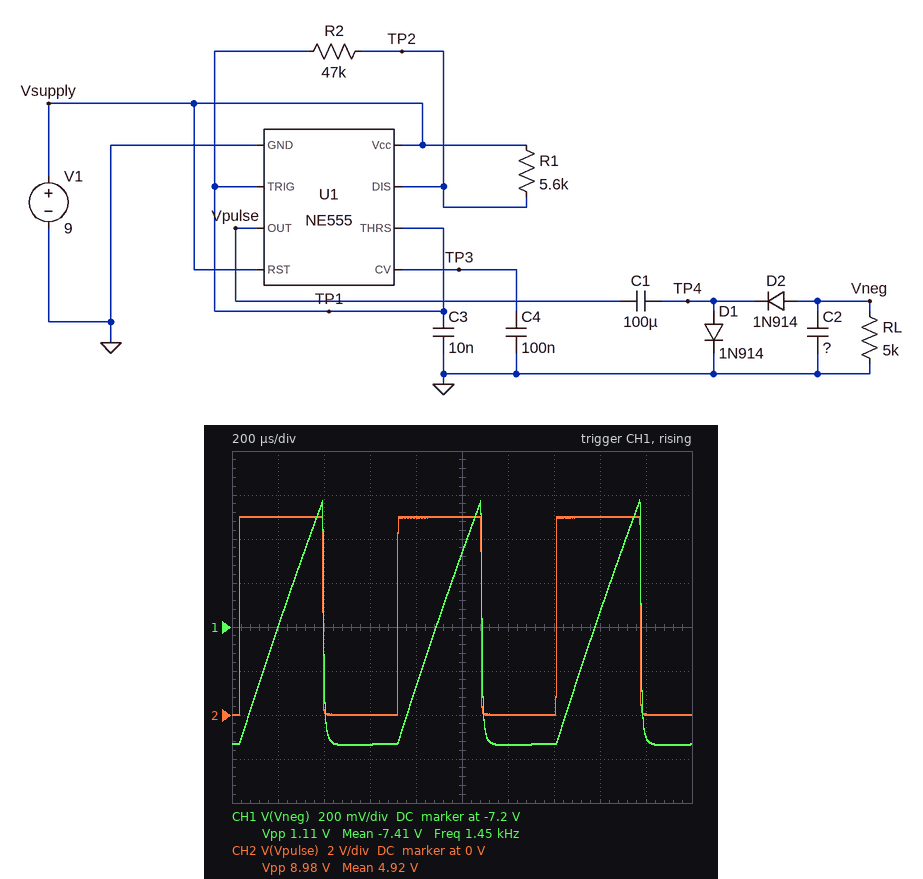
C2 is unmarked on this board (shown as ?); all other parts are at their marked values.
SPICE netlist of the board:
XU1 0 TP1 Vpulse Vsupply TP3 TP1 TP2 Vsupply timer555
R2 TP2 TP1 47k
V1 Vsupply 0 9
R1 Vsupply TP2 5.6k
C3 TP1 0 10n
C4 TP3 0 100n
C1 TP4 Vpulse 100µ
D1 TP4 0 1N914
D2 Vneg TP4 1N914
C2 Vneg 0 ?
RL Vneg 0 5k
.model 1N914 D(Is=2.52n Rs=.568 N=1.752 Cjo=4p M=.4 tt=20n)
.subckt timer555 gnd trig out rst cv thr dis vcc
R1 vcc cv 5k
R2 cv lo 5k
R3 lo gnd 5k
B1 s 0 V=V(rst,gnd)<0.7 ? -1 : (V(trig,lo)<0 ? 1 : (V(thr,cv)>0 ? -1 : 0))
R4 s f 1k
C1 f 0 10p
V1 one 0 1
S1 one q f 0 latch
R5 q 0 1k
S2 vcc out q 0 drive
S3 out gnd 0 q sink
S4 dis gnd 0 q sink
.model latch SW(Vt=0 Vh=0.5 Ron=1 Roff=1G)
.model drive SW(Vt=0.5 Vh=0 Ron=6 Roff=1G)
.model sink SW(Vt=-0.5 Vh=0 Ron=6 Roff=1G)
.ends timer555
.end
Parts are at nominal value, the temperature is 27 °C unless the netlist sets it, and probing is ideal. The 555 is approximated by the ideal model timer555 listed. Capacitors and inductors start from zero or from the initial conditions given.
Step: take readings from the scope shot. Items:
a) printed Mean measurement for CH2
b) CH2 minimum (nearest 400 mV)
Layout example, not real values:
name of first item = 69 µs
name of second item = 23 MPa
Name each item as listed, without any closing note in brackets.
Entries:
printed Mean measurement for CH2 = 4.92 V
CH2 minimum = 0 V
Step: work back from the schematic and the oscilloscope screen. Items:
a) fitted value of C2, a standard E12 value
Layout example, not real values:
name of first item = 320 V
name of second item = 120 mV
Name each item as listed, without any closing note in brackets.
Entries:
fitted value of C2, a standard E12 value = 470 nF
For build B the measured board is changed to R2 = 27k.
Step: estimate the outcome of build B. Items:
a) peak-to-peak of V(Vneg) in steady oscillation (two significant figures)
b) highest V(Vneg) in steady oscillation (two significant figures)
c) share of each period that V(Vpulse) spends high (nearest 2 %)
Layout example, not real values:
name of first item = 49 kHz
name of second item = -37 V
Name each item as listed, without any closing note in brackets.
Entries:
peak-to-peak of V(Vneg) in steady oscillation = 710 mV
highest V(Vneg) in steady oscillation = -7.0 V
share of each period that V(Vpulse) spends high = 54 %
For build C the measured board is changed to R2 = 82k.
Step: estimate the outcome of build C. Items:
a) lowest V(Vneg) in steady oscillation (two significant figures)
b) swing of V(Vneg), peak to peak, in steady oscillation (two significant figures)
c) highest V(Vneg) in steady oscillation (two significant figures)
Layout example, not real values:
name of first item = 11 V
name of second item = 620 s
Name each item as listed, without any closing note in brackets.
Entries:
lowest V(Vneg) in steady oscillation = -7.7 V
swing of V(Vneg), peak to peak, in steady oscillation = 1.8 V
highest V(Vneg) in steady oscillation = -6.0 V
